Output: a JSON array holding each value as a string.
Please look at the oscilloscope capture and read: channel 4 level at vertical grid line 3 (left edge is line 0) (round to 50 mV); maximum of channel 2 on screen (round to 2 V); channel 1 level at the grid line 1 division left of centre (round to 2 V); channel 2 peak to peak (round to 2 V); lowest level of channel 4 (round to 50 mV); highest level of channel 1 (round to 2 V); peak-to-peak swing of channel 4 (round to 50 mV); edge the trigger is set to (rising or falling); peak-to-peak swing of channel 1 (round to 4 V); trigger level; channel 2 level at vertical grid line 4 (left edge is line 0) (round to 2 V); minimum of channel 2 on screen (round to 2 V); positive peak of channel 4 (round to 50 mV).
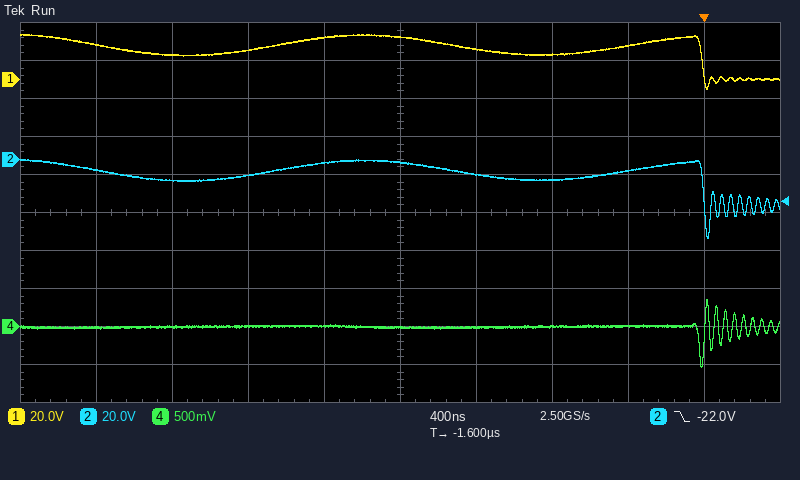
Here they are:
["0 mV", "0 V", "22 V", "42 V", "-550 mV", "24 V", "900 mV", "falling", "28 V", "-22.0 V", "-2 V", "-42 V", "350 mV"]
